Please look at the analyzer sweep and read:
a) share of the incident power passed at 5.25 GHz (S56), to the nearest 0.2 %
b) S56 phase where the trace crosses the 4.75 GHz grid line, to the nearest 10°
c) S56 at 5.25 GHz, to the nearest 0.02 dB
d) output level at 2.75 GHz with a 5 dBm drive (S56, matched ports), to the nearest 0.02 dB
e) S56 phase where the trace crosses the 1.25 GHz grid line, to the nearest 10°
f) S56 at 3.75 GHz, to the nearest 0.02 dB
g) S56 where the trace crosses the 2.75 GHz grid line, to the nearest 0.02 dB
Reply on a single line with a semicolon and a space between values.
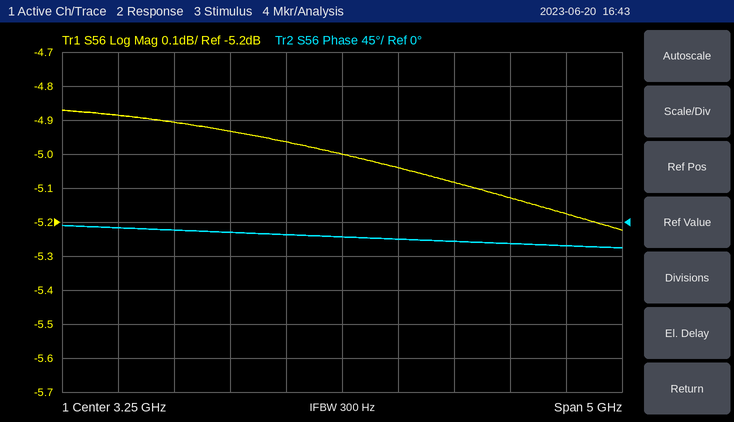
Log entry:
30.4 %; -30°; -5.18 dB; 0.04 dBm; -10°; -5.04 dB; -4.96 dB
